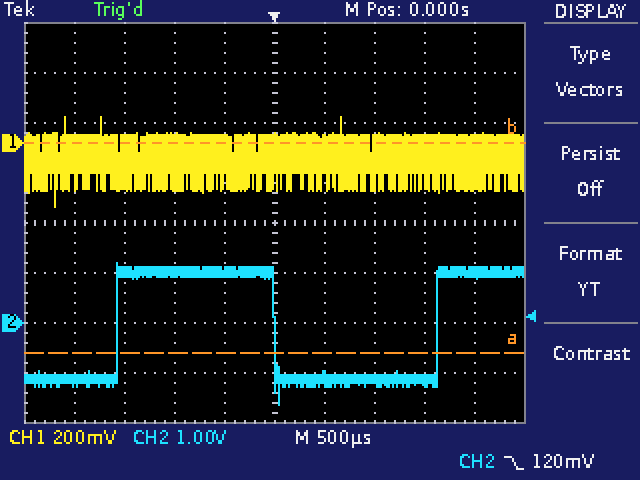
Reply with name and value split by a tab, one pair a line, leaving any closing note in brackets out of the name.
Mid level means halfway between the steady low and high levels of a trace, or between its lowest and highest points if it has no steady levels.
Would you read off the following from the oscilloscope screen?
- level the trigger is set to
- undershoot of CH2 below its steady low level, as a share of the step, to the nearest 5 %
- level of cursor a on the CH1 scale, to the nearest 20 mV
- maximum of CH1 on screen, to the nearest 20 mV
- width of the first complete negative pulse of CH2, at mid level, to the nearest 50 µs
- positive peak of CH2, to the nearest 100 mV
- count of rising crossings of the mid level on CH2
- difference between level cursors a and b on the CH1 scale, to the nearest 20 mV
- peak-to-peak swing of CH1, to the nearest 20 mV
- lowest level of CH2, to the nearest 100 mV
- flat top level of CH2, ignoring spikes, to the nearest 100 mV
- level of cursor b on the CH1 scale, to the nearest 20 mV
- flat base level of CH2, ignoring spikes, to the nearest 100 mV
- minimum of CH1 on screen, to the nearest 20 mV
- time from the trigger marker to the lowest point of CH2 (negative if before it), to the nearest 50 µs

level the trigger is set to	120 mV
undershoot of CH2 below its steady low level, as a share of the step, to the nearest 5 %	25 %
level of cursor a on the CH1 scale, to the nearest 20 mV	-840 mV
maximum of CH1 on screen, to the nearest 20 mV	100 mV
width of the first complete negative pulse of CH2, at mid level, to the nearest 50 µs	1.65 ms
positive peak of CH2, to the nearest 100 mV	1.2 V
count of rising crossings of the mid level on CH2	2
difference between level cursors a and b on the CH1 scale, to the nearest 20 mV	840 mV
peak-to-peak swing of CH1, to the nearest 20 mV	360 mV
lowest level of CH2, to the nearest 100 mV	-1.6 V
flat top level of CH2, ignoring spikes, to the nearest 100 mV	1.0 V
level of cursor b on the CH1 scale, to the nearest 20 mV	0 mV
flat base level of CH2, ignoring spikes, to the nearest 100 mV	-1.1 V
minimum of CH1 on screen, to the nearest 20 mV	-260 mV
time from the trigger marker to the lowest point of CH2 (negative if before it), to the nearest 50 µs	+50 µs
